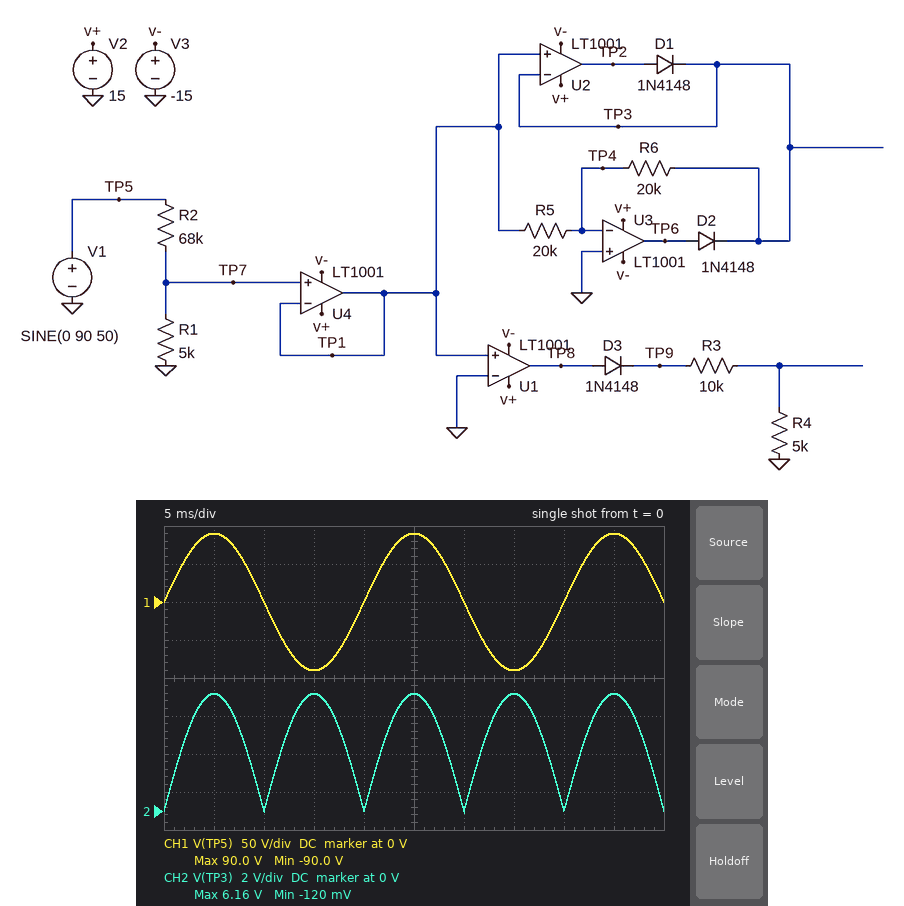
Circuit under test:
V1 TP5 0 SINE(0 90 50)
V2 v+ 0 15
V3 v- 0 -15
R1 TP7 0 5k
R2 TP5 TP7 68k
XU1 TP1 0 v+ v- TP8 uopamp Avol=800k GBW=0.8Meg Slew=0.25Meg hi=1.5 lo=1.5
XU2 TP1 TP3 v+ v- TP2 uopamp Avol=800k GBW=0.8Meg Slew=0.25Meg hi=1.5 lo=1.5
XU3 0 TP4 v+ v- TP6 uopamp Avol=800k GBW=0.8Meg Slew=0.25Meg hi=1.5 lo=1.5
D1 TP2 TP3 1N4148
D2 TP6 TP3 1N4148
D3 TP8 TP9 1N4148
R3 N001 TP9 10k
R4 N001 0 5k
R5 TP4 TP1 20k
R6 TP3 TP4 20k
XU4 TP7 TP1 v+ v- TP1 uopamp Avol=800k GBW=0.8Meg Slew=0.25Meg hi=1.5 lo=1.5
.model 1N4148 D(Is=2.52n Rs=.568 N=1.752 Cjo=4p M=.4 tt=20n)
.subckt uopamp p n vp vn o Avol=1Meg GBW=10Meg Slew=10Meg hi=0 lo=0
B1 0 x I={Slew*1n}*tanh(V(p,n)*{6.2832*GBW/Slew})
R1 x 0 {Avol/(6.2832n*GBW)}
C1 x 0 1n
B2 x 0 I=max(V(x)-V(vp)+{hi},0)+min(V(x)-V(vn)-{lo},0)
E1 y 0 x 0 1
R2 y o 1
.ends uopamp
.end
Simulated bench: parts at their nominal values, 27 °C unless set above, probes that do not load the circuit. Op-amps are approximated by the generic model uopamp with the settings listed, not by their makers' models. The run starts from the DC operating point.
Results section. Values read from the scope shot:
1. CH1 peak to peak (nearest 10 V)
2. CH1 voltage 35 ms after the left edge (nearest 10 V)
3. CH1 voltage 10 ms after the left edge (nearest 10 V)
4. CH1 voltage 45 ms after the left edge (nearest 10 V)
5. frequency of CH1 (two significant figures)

180 V
-90 V
0 V
90 V
50 Hz
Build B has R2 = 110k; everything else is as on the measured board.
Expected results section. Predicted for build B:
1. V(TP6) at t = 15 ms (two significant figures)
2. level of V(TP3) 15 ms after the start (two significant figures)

4.4 V
3.9 V
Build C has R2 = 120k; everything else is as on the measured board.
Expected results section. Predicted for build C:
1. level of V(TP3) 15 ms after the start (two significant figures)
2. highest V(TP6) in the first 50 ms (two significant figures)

3.6 V
4.1 V
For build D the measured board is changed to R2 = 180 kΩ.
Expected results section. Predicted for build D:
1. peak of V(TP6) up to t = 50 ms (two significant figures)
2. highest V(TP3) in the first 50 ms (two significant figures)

2.9 V
2.4 V
